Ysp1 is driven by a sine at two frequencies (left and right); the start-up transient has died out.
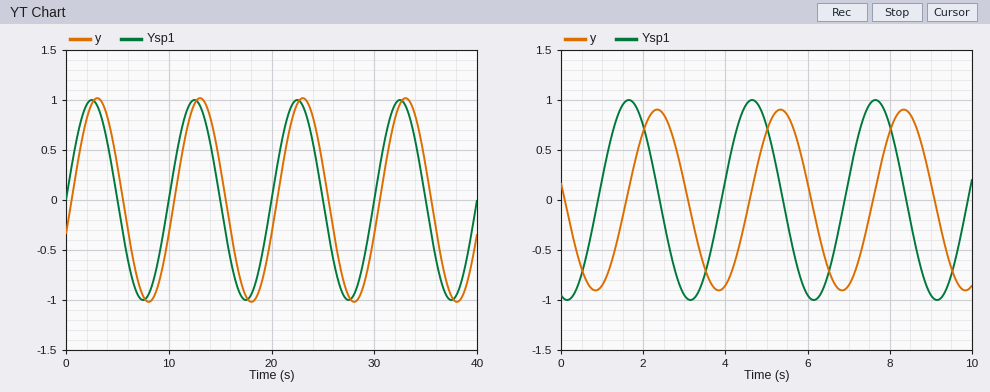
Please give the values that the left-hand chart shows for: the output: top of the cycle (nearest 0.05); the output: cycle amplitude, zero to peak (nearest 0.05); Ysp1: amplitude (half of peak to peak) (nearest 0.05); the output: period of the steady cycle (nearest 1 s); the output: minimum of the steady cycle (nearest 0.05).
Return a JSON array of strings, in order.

["1.00", "1.00", "1.00", "10 s", "-1.00"]
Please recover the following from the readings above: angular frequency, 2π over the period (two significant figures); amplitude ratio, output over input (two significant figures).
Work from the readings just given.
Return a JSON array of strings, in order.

["0.63 rad/s", "1.0"]
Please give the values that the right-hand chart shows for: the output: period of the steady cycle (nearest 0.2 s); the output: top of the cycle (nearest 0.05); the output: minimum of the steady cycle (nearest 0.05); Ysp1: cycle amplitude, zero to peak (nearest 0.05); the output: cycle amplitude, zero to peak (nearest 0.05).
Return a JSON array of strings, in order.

["3.0 s", "0.90", "-0.90", "1.00", "0.90"]
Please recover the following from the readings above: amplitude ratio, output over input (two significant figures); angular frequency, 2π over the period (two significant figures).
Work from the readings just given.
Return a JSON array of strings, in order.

["0.90", "2.1 rad/s"]
